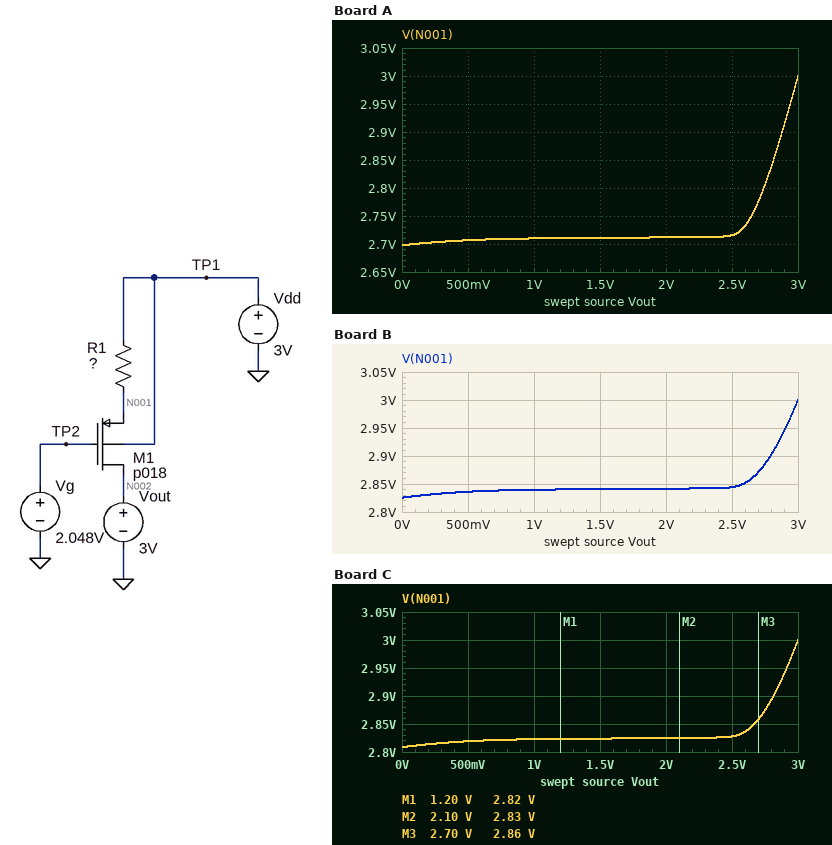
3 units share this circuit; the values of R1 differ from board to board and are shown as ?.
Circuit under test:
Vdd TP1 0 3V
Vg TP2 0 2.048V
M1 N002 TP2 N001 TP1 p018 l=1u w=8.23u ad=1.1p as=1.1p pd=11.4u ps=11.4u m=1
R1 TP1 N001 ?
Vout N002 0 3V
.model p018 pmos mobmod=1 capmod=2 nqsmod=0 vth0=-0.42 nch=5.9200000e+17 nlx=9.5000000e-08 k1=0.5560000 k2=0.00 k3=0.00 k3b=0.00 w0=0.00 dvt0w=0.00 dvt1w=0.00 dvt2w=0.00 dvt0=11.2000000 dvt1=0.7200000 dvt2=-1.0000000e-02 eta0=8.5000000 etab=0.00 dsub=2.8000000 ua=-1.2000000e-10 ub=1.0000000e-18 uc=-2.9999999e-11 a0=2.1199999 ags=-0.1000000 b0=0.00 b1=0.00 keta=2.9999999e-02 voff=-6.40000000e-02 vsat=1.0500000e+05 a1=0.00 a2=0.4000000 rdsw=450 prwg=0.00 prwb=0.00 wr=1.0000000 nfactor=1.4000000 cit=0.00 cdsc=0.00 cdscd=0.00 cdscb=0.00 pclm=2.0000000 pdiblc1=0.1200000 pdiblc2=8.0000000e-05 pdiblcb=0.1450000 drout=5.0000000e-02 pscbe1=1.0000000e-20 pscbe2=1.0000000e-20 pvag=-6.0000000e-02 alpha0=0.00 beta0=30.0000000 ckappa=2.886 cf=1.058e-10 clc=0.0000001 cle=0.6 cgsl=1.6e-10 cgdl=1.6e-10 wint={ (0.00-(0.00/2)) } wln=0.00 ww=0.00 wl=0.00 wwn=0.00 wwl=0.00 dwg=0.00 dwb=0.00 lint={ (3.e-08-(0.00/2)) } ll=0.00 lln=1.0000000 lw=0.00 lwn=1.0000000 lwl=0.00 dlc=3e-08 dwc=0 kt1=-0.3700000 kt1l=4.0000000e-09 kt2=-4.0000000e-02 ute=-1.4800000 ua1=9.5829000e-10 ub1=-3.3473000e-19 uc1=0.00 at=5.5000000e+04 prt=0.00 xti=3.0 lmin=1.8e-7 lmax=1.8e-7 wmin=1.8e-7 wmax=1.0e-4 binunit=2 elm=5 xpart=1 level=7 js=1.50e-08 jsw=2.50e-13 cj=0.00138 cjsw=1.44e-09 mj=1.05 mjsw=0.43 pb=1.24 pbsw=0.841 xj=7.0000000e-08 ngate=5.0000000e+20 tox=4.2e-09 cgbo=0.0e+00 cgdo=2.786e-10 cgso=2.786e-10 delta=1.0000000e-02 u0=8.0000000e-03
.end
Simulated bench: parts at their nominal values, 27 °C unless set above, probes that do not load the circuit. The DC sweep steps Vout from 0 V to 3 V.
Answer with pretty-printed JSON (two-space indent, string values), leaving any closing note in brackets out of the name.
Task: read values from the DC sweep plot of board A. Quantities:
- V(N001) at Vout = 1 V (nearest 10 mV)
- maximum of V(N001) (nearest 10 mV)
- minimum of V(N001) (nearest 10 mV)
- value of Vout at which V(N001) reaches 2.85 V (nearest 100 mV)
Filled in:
{
  "V(N001) at Vout = 1 V": "2.71 V",
  "maximum of V(N001)": "3.00 V",
  "minimum of V(N001)": "2.70 V",
  "value of Vout at which V(N001) reaches 2.85 V": "2.8 V"
}
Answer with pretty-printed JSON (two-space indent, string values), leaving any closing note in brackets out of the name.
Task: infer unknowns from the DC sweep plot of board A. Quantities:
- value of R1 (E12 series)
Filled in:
{
  "value of R1": "39 kΩ"
}
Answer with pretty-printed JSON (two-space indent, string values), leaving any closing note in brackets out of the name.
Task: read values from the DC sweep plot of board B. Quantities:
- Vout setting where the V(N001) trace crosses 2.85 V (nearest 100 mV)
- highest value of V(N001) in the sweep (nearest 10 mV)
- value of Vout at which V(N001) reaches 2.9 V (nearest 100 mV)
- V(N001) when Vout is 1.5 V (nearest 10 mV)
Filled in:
{
  "Vout setting where the V(N001) trace crosses 2.85 V": "2.6 V",
  "highest value of V(N001) in the sweep": "3.00 V",
  "value of Vout at which V(N001) reaches 2.9 V": "2.8 V",
  "V(N001) when Vout is 1.5 V": "2.84 V"
}
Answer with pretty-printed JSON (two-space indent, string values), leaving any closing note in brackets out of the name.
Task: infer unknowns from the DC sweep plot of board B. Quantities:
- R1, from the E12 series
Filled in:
{
  "R1, from the E12 series": "8.2 kΩ"
}
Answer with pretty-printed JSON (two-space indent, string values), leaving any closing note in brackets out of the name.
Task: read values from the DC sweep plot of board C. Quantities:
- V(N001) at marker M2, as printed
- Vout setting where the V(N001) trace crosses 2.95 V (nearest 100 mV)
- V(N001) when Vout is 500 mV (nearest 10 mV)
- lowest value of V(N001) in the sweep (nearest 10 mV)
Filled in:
{
  "V(N001) at marker M2, as printed": "2.83 V",
  "Vout setting where the V(N001) trace crosses 2.95 V": "2.9 V",
  "V(N001) when Vout is 500 mV": "2.82 V",
  "lowest value of V(N001) in the sweep": "2.81 V"
}
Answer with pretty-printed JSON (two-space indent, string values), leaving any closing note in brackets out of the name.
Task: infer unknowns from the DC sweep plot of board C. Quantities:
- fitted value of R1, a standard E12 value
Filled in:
{
  "fitted value of R1, a standard E12 value": "10 kΩ"
}
